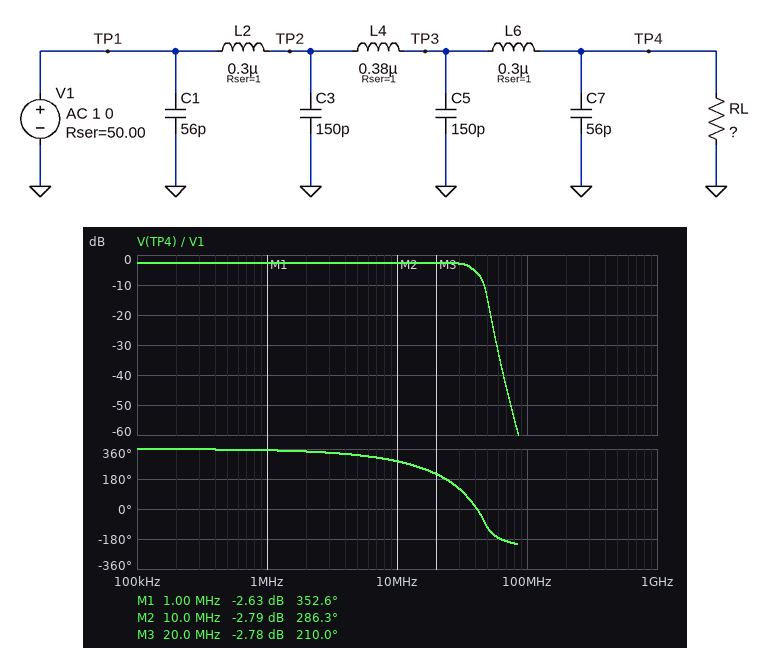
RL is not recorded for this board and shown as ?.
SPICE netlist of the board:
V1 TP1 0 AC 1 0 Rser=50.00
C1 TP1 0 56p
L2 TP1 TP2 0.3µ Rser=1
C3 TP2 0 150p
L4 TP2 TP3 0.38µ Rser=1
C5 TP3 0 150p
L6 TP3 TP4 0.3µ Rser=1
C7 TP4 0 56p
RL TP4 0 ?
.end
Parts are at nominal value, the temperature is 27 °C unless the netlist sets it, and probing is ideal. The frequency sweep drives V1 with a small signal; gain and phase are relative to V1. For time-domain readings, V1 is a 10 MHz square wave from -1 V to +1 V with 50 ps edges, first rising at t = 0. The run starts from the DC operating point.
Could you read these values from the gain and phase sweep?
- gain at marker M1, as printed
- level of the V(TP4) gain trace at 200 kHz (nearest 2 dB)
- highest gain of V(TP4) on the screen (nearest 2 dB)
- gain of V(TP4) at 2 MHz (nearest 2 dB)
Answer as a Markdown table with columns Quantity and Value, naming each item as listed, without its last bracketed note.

| Quantity | Value |
|---|---|
| gain at marker M1, as printed | -2.63 dB |
| level of the V(TP4) gain trace at 200 kHz | -2 dB |
| highest gain of V(TP4) on the screen | -2 dB |
| gain of V(TP4) at 2 MHz | -2 dB |
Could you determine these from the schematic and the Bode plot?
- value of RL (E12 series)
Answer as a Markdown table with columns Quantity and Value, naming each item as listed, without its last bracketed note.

| Quantity | Value |
|---|---|
| value of RL | 150 Ω |
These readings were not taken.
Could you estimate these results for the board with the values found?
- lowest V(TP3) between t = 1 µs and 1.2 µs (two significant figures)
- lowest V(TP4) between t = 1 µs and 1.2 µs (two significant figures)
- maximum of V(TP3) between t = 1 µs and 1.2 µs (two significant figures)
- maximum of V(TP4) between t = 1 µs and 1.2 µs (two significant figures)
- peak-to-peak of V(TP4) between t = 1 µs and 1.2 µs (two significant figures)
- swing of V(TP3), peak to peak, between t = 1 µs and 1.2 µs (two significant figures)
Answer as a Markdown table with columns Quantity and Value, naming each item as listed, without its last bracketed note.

| Quantity | Value |
|---|---|
| lowest V(TP3) between t = 1 µs and 1.2 µs | -750 mV |
| lowest V(TP4) between t = 1 µs and 1.2 µs | -960 mV |
| maximum of V(TP3) between t = 1 µs and 1.2 µs | 750 mV |
| maximum of V(TP4) between t = 1 µs and 1.2 µs | 960 mV |
| peak-to-peak of V(TP4) between t = 1 µs and 1.2 µs | 1.9 V |
| swing of V(TP3), peak to peak, between t = 1 µs and 1.2 µs | 1.5 V |
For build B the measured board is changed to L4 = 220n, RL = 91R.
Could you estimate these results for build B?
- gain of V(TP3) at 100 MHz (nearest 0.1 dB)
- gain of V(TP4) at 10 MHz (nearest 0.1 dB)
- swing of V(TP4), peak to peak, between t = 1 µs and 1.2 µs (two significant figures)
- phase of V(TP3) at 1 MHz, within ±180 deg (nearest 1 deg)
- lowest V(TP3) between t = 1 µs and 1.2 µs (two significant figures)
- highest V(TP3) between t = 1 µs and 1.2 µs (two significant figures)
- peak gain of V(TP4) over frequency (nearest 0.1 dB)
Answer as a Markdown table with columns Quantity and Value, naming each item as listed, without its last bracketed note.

| Quantity | Value |
|---|---|
| gain of V(TP3) at 100 MHz | -49.7 dB |
| gain of V(TP4) at 10 MHz | -4.4 dB |
| swing of V(TP4), peak to peak, between t = 1 µs and 1.2 µs | 1.6 V |
| phase of V(TP3) at 1 MHz, within ±180 deg | -6 deg |
| lowest V(TP3) between t = 1 µs and 1.2 µs | -730 mV |
| highest V(TP3) between t = 1 µs and 1.2 µs | 730 mV |
| peak gain of V(TP4) over frequency | -4.0 dB |
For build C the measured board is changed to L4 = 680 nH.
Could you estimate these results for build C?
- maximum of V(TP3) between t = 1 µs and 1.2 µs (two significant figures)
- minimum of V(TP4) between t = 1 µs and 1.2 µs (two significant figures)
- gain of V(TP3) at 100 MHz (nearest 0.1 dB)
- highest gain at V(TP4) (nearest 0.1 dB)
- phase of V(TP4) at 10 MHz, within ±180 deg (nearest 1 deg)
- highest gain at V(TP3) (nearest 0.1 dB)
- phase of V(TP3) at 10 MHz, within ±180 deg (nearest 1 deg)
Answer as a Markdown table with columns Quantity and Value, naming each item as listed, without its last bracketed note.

| Quantity | Value |
|---|---|
| maximum of V(TP3) between t = 1 µs and 1.2 µs | 870 mV |
| minimum of V(TP4) between t = 1 µs and 1.2 µs | -930 mV |
| gain of V(TP3) at 100 MHz | -60.6 dB |
| highest gain at V(TP4) | -2.0 dB |
| phase of V(TP4) at 10 MHz, within ±180 deg | -84 deg |
| highest gain at V(TP3) | -2.5 dB |
| phase of V(TP3) at 10 MHz, within ±180 deg | -76 deg |
